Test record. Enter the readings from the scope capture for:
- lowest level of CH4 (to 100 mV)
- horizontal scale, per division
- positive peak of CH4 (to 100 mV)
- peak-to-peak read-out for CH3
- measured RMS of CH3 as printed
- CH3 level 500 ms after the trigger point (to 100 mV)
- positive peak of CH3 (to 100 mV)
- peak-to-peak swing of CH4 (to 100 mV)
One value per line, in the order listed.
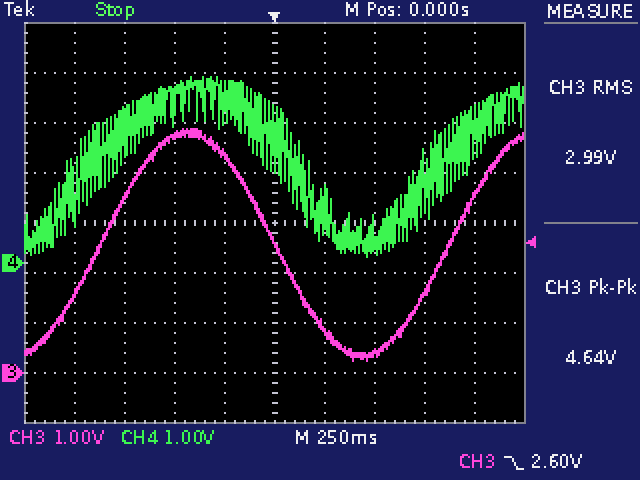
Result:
100 mV
250 ms
3.7 V
4.64 V
2.99 V
400 mV
4.9 V
3.6 V
